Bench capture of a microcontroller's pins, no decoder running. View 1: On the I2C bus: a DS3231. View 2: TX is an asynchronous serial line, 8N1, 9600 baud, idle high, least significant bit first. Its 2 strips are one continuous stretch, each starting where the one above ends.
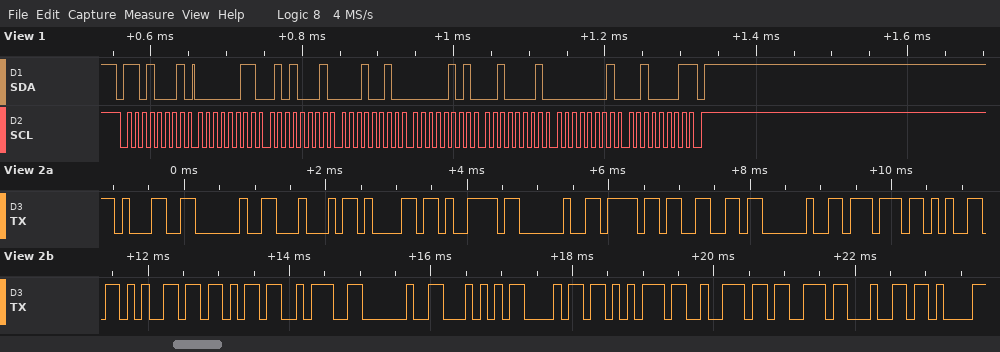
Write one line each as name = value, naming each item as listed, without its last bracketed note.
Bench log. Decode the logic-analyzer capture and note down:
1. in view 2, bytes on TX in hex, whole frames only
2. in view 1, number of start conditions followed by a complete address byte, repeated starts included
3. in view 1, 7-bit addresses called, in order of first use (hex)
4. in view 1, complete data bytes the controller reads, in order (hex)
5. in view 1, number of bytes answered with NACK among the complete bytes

in view 2, bytes on TX in hex, whole frames only = 31 20 44 61 79 20 6F 66 20 77 65 65 6B 3A 20 54 68 75 72 73 64
in view 1, number of start conditions followed by a complete address byte, repeated starts included = 1
in view 1, 7-bit addresses called, in order of first use = 0x68
in view 1, complete data bytes the controller reads, in order = 03 51 12 05 21 01 21
in view 1, number of bytes answered with NACK among the complete bytes = 1
